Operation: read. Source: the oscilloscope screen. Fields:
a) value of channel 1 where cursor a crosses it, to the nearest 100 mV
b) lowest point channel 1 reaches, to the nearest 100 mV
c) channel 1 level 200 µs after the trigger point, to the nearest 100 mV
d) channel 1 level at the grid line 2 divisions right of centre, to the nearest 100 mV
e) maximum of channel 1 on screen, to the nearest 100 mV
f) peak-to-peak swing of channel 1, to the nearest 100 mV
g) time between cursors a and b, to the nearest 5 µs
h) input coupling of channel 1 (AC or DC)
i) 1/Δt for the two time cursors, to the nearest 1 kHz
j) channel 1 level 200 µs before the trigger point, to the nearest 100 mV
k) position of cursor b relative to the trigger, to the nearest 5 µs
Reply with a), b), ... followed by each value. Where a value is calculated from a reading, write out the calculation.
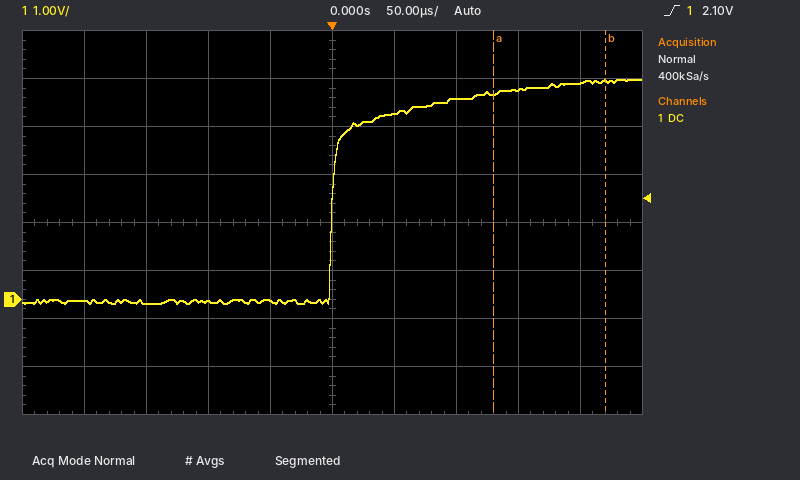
a) 4.3 V
b) -100 mV
c) 4.5 V
d) 4.2 V
e) 4.6 V
f) 4.6 V − (-100 mV) = 4.7 V
g) 90 µs
h) DC
i) 1 / 90 µs ≈ 11 kHz
j) 0.0 V
k) +220 µs
